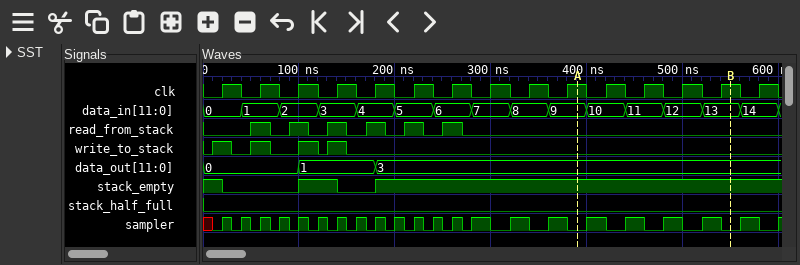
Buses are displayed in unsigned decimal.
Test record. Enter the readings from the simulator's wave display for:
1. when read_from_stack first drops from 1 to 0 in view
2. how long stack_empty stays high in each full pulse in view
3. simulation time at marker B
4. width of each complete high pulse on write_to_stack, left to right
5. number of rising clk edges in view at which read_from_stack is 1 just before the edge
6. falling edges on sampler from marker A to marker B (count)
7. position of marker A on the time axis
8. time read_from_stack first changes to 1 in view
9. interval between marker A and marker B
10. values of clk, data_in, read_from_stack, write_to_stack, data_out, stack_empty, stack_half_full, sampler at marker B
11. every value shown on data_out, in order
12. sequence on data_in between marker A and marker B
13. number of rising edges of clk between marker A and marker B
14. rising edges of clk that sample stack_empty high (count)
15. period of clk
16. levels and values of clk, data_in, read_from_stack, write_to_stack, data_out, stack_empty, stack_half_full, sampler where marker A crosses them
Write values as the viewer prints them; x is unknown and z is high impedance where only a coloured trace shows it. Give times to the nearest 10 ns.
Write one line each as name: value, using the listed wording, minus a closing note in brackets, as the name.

when read_from_stack first drops from 1 to 0 in view: 70 ns
how long stack_empty stays high in each full pulse in view: 40 ns
simulation time at marker B: 550 ns
width of each complete high pulse on write_to_stack, left to right: 20 ns, 20 ns, 20 ns, 20 ns
number of rising clk edges in view at which read_from_stack is 1 just before the edge: 6
falling edges on sampler from marker A to marker B: 4
position of marker A on the time axis: 390 ns
time read_from_stack first changes to 1 in view: 50 ns
interval between marker A and marker B: 160 ns
values of clk, data_in, read_from_stack, write_to_stack, data_out, stack_empty, stack_half_full, sampler at marker B: clk=1, data_in=13, read_from_stack=0, write_to_stack=0, data_out=3, stack_empty=1, stack_half_full=0, sampler=0
every value shown on data_out, in order: 0, 1, 3
sequence on data_in between marker A and marker B: 9, 10, 11, 12, 13
number of rising edges of clk between marker A and marker B: 4
rising edges of clk that sample stack_empty high: 12
period of clk: 40 ns
levels and values of clk, data_in, read_from_stack, write_to_stack, data_out, stack_empty, stack_half_full, sampler where marker A crosses them: clk=1, data_in=9, read_from_stack=0, write_to_stack=0, data_out=3, stack_empty=1, stack_half_full=0, sampler=0
